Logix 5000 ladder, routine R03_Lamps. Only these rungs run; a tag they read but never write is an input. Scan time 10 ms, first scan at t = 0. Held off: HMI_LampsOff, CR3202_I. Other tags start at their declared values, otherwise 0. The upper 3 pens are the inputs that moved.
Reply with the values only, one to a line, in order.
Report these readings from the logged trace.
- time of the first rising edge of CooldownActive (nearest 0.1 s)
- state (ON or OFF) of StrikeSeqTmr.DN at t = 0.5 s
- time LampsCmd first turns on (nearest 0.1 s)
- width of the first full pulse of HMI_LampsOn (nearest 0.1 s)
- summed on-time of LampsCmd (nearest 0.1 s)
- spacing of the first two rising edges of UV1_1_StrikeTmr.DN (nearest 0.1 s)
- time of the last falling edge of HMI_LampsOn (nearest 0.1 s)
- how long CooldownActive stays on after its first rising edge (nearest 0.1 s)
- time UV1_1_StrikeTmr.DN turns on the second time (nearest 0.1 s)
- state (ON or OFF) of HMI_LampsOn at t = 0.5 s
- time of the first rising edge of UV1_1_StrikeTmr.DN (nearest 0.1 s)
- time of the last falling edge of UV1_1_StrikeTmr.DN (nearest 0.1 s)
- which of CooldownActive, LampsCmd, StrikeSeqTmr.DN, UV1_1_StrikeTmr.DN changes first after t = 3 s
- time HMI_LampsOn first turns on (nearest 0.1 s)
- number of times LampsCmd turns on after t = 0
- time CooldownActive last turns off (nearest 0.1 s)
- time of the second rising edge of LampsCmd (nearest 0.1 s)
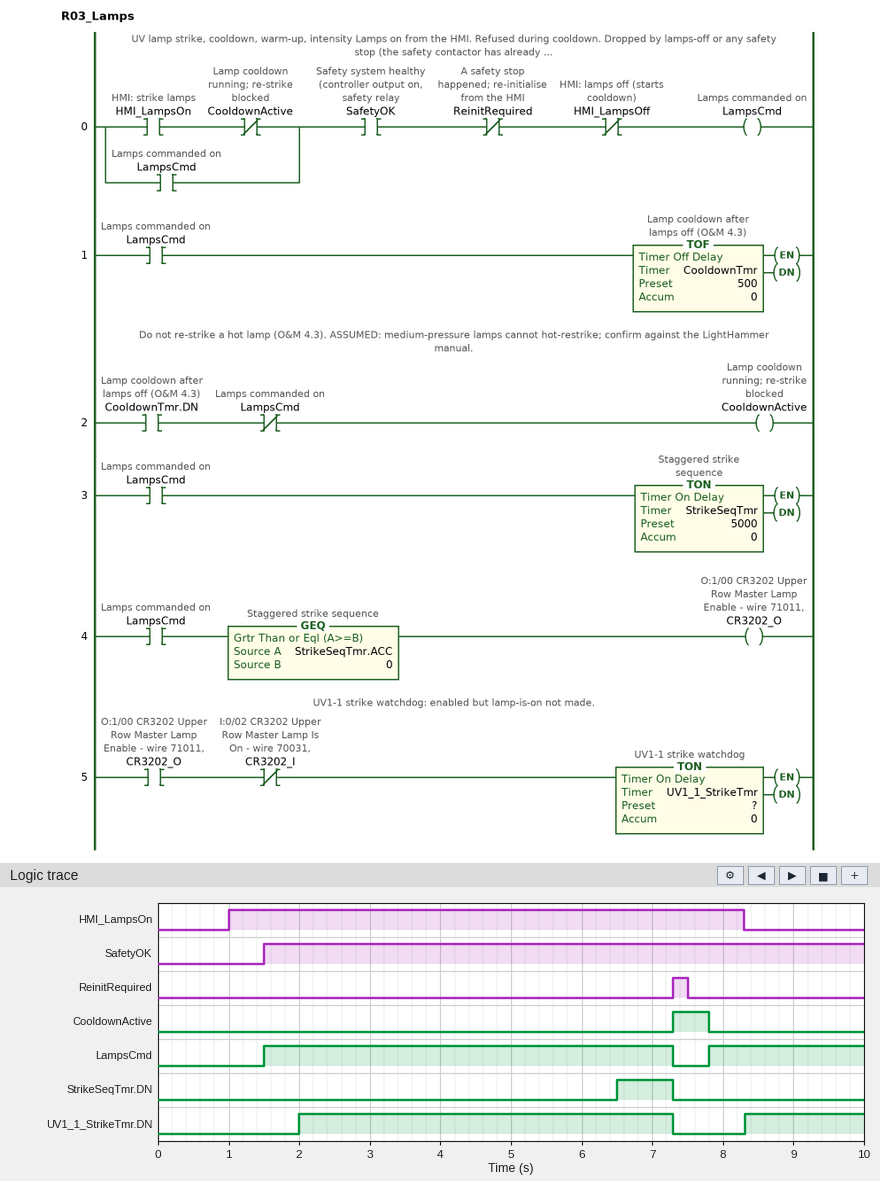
7.3 s
OFF
1.5 s
7.3 s
8.0 s
6.3 s
8.3 s
0.5 s
8.3 s
OFF
2.0 s
7.3 s
StrikeSeqTmr.DN
1.0 s
2
7.8 s
7.8 s
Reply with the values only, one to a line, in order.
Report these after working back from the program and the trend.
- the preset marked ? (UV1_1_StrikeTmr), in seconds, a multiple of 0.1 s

0.5 s
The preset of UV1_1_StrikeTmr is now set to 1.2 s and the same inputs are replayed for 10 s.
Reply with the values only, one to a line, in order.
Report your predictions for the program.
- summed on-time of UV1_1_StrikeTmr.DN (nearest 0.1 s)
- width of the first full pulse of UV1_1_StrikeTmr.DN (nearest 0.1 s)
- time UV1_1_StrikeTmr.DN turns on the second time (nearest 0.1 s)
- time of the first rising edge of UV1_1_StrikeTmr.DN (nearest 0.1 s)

5.6 s
4.6 s
9.0 s
2.7 s
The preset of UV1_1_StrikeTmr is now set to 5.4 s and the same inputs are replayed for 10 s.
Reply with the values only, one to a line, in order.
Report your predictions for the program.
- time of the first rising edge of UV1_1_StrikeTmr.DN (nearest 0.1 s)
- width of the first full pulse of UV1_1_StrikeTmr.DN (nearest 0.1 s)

6.9 s
0.4 s
